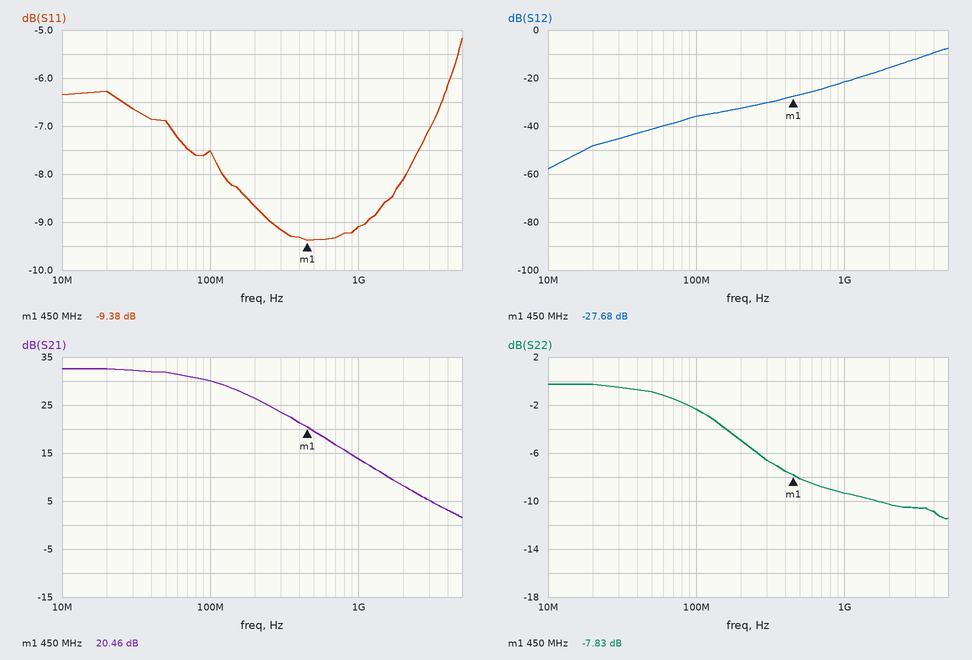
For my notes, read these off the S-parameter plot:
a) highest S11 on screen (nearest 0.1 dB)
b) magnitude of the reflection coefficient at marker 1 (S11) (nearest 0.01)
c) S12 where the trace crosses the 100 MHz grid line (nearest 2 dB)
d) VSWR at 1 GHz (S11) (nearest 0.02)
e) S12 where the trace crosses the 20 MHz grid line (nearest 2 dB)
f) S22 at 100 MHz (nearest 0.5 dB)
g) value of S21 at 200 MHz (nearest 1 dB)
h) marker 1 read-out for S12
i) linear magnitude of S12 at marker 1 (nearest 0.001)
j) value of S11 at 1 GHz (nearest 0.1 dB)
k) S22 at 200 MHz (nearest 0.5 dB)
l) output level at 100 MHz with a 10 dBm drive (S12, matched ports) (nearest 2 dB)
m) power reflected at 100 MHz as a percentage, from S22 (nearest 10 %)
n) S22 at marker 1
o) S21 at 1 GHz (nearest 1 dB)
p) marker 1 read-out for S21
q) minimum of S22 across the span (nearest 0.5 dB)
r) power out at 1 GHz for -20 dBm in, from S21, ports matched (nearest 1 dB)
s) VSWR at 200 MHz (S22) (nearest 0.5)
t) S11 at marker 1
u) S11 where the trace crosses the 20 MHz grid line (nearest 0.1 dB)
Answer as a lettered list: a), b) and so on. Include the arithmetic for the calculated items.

a) -5.2 dB
b) 10^(-9.38/20) ≈ 0.34
c) -36 dB
d) |Γ| = 10^(-9.1/20) = 0.3508; VSWR = (1 + 0.3508)/(1 − 0.3508) ≈ 2.08
e) -48 dB
f) -2.5 dB
g) 26 dB
h) -27.68 dB
i) 10^(-27.68/20) ≈ 0.041
j) -9.1 dB
k) -5.0 dB
l) 10 dBm + (-36 dB) = -26 dBm
m) 10^(-2.5/10) ≈ 56.2 %, so 60 % to the nearest 10 %
n) -7.83 dB
o) 14 dB
p) 20.46 dB
q) -11.5 dB
r) -20 dBm + (14 dB) = -6 dBm
s) |Γ| = 10^(-5/20) = 0.5623; VSWR = (1 + 0.5623)/(1 − 0.5623) ≈ 3.57, so 3.5 to the nearest 0.5
t) -9.38 dB
u) -6.3 dB
